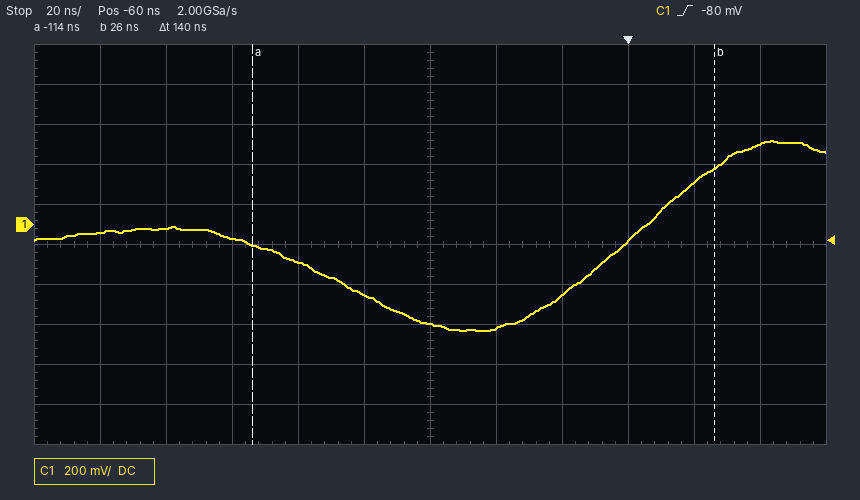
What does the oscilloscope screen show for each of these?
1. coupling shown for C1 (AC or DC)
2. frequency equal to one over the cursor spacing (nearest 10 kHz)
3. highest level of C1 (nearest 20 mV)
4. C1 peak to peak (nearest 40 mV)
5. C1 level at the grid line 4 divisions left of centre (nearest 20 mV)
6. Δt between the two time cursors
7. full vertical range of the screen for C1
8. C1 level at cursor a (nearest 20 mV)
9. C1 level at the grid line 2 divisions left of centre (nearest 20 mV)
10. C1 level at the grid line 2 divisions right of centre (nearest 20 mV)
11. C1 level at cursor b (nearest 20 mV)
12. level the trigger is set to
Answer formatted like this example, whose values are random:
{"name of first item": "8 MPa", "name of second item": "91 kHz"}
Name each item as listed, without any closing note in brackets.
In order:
{"coupling shown for C1": "DC", "frequency equal to one over the cursor spacing": "7.14 MHz", "highest level of C1": "420 mV", "C1 peak to peak": "960 mV", "C1 level at the grid line 4 divisions left of centre": "-20 mV", "Δt between the two time cursors": "140 ns", "full vertical range of the screen for C1": "2 V", "C1 level at cursor a": "-100 mV", "C1 level at the grid line 2 divisions left of centre": "-180 mV", "C1 level at the grid line 2 divisions right of centre": "-360 mV", "C1 level at cursor b": "280 mV", "level the trigger is set to": "-80 mV"}
